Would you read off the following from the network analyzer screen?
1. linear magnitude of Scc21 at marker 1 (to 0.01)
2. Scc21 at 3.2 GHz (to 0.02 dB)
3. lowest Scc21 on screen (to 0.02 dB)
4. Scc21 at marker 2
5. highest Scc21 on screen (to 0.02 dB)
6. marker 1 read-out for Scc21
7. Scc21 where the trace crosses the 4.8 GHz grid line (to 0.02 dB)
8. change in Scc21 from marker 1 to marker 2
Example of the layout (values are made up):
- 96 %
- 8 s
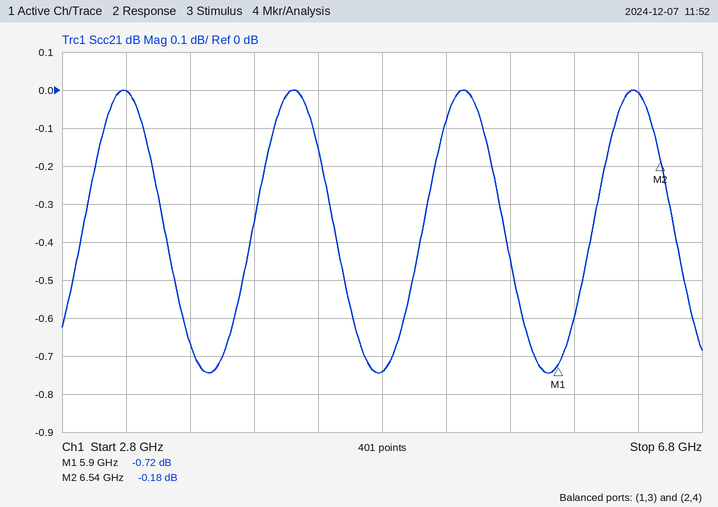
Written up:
- 0.92
- 0.00 dB
- -0.74 dB
- -0.18 dB
- 0.00 dB
- -0.72 dB
- -0.74 dB
- 0.54 dB
